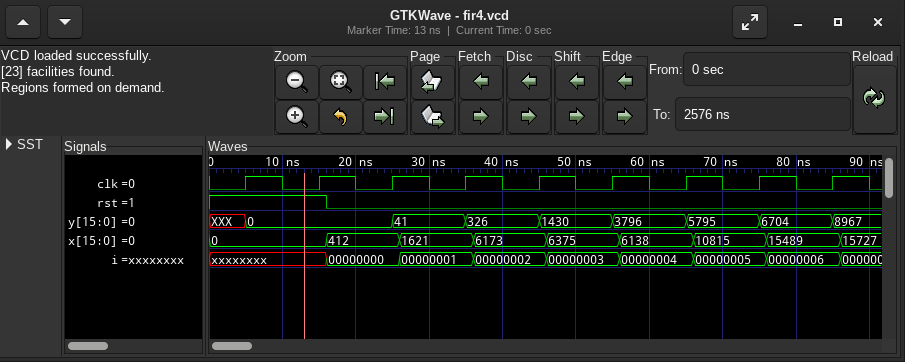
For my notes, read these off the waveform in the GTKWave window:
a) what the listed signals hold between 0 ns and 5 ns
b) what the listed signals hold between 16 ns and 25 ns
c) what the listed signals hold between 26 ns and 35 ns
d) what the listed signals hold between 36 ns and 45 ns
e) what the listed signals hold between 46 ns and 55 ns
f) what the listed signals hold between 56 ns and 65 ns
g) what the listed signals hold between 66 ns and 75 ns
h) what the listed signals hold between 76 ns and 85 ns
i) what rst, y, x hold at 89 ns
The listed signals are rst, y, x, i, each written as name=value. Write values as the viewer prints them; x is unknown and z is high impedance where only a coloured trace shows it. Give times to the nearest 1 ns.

rst=1, y=XXX, x=0, i=xxxxxxxx
rst=0, y=0, x=412, i=00000000
rst=0, y=41, x=1621, i=00000001
rst=0, y=326, x=6173, i=00000002
rst=0, y=1430, x=6375, i=00000003
rst=0, y=3796, x=6138, i=00000004
rst=0, y=5795, x=10815, i=00000005
rst=0, y=6704, x=15489, i=00000006
rst=0, y=8967, x=15727
